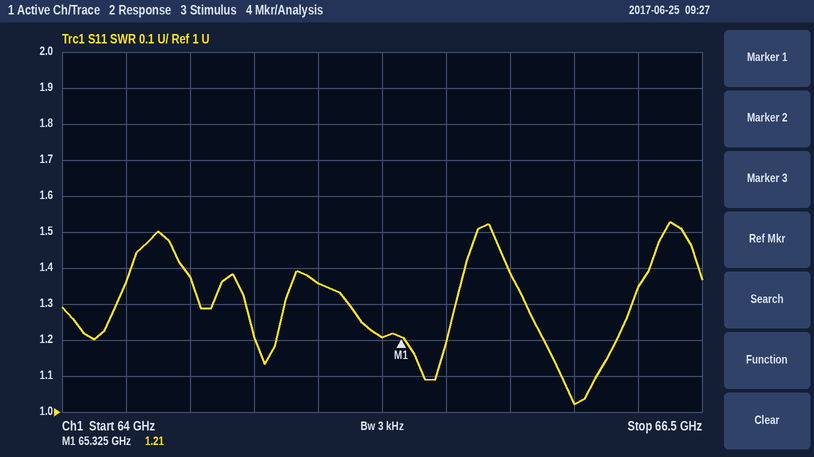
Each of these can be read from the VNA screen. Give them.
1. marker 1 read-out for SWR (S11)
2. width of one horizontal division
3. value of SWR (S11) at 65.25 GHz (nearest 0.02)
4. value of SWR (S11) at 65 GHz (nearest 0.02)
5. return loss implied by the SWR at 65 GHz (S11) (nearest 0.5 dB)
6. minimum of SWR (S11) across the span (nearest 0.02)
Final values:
1.21
250 MHz
1.20
1.36
16.5 dB
1.02
